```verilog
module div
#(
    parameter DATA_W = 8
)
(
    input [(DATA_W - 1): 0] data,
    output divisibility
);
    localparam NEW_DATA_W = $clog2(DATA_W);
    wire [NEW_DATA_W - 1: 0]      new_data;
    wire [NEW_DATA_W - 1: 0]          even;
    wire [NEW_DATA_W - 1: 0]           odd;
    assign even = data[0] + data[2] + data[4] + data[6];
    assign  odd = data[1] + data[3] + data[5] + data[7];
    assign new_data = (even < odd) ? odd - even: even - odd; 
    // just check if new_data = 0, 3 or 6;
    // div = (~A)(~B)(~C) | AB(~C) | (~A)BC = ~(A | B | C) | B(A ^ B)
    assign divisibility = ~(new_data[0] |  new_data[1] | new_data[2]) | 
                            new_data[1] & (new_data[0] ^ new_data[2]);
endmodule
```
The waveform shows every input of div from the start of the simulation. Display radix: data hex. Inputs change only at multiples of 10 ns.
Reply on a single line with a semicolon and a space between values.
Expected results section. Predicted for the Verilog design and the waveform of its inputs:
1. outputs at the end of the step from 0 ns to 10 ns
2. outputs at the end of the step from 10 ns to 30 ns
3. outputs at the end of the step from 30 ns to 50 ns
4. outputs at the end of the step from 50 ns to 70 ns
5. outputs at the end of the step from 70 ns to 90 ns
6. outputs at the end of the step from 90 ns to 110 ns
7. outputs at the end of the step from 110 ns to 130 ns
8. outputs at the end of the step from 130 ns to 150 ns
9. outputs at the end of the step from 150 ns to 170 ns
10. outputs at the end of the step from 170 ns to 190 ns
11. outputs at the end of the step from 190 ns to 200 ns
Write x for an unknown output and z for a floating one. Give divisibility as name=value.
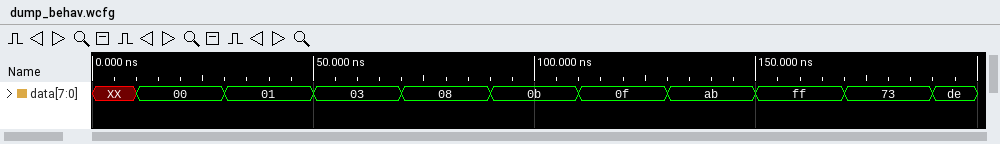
divisibility=x; divisibility=1; divisibility=0; divisibility=1; divisibility=0; divisibility=0; divisibility=1; divisibility=1; divisibility=1; divisibility=0; divisibility=1
